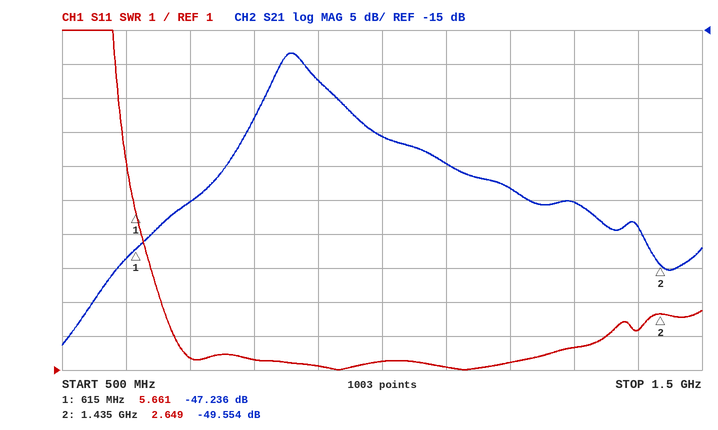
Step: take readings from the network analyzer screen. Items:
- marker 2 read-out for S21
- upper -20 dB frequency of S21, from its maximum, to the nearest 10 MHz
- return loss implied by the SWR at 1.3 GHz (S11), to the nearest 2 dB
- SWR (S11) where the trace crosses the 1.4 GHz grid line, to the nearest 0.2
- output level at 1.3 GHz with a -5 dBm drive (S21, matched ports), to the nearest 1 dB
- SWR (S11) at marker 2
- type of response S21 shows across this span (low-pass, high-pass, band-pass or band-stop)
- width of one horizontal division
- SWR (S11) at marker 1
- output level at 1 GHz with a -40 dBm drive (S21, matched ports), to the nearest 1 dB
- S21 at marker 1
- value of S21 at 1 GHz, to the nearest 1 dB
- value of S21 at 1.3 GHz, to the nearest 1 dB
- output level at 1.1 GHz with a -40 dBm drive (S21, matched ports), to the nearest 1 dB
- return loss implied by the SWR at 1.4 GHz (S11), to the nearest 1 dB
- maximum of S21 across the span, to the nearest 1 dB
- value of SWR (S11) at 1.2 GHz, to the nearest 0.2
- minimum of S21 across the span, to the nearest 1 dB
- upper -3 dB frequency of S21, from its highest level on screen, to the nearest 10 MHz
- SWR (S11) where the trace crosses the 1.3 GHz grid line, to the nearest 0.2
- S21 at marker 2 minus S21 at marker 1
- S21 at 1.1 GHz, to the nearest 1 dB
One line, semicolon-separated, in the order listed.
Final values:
-49.554 dB; 1.20 GHz; 12 dB; 2.2; -45 dBm; 2.649; band-pass; 100 MHz; 5.661; -71 dBm; -47.236 dB; -31 dB; -40 dB; -75 dBm; 9 dB; -18 dB; 1.2; -61 dB; 890 MHz; 1.6; -2.318 dB; -35 dB
